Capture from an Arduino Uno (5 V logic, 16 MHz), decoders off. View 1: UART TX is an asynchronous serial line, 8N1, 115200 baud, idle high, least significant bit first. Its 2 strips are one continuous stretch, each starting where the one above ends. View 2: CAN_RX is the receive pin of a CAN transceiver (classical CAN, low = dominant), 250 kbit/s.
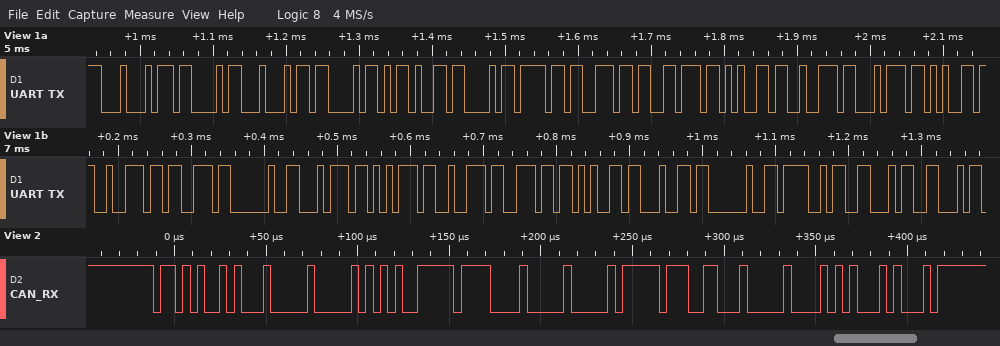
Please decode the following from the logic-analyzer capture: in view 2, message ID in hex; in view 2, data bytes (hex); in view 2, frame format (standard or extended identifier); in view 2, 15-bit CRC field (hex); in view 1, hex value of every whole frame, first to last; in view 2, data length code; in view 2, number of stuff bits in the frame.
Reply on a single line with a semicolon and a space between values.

0x6A5; 00 A9 FF 08 00 FF 31 00; standard; 0x2A28; 44 43 44 43 2D 43 6F 6E 76 65 72 74 65 72 73 20 74 75 72 6E 65 64 20 4F 46 46; 8; 7
